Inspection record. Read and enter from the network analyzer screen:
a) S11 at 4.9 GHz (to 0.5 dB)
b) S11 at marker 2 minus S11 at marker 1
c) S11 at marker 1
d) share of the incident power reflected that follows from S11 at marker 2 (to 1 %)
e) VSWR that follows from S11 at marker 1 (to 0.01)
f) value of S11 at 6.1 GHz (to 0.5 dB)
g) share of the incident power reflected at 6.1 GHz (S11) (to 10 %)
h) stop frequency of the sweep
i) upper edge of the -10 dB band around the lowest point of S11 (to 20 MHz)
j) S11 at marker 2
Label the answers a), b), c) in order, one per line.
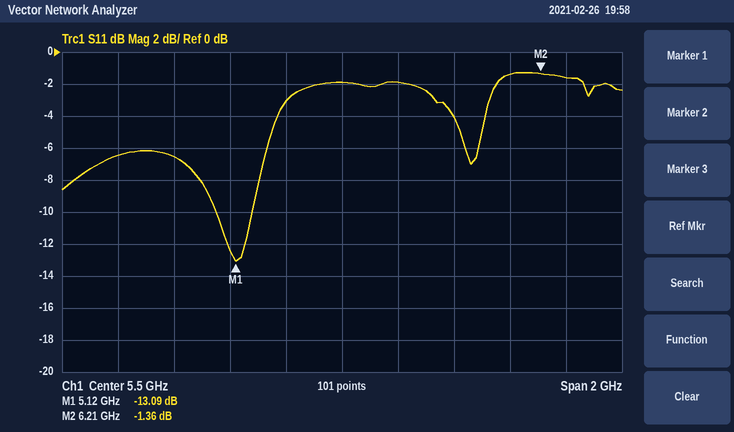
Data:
a) -6.5 dB
b) 11.73 dB
c) -13.09 dB
d) 73 %
e) 1.57
f) -1.5 dB
g) 70 %
h) 6.5 GHz
i) 5.18 GHz
j) -1.36 dB
